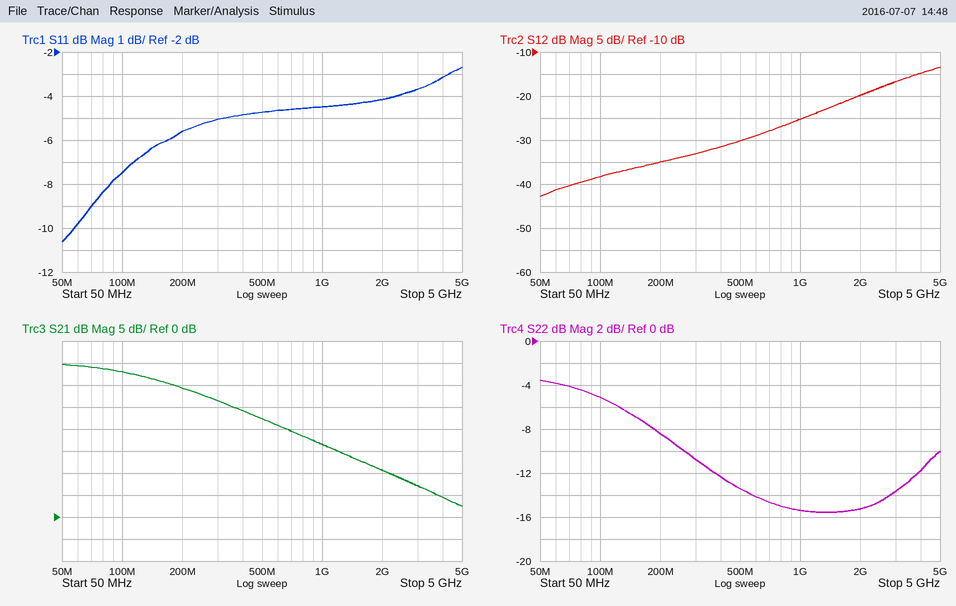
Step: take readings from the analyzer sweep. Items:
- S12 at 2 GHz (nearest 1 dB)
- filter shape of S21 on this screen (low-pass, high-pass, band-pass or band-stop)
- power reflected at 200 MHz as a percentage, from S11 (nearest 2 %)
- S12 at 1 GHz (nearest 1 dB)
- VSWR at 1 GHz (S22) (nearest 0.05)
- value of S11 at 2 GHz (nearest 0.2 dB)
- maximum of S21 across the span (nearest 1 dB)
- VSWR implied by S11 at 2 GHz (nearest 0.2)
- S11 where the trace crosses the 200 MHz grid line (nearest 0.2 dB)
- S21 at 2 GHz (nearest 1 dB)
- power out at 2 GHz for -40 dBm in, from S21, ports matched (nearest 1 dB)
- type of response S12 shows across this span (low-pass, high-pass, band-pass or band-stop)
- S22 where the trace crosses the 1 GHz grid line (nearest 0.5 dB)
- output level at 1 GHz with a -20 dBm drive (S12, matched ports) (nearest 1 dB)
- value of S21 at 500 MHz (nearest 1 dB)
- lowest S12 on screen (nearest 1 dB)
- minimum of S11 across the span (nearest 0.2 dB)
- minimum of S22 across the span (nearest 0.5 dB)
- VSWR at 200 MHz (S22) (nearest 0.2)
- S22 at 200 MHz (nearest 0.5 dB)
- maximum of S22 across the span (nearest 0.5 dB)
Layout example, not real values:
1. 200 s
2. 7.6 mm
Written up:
1. -20 dB
2. low-pass
3. 28 %
4. -25 dB
5. 1.40
6. -4.2 dB
7. 35 dB
8. 4.2
9. -5.6 dB
10. 11 dB
11. -29 dBm
12. high-pass
13. -15.5 dB
14. -45 dBm
15. 22 dB
16. -43 dB
17. -10.6 dB
18. -15.5 dB
19. 2.2
20. -8.5 dB
21. -3.5 dB
